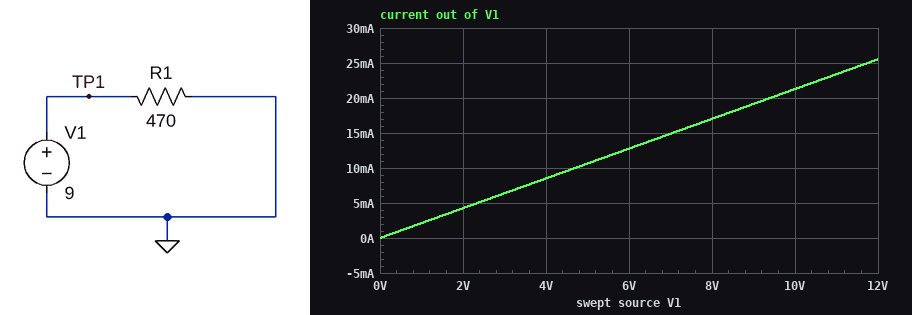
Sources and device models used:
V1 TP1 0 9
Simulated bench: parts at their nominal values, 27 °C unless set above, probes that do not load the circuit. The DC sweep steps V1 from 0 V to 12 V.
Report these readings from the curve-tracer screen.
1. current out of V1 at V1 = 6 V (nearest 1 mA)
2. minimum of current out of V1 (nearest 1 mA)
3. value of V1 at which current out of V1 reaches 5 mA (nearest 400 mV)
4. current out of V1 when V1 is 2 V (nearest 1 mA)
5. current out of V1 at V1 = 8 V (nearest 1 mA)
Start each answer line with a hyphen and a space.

- 13 mA
- 0 A
- 2.4 V
- 4 mA
- 17 mA
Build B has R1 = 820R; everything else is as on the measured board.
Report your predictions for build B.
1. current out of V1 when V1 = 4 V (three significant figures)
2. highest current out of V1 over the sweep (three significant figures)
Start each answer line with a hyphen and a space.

- 4.88 mA
- 14.6 mA
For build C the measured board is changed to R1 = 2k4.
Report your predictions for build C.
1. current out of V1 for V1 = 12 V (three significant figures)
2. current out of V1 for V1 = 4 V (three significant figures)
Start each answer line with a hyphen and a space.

- 5.00 mA
- 1.67 mA
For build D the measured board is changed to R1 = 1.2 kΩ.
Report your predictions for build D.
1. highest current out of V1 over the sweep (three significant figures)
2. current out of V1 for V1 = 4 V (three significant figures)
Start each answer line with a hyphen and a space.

- 10.0 mA
- 3.33 mA
